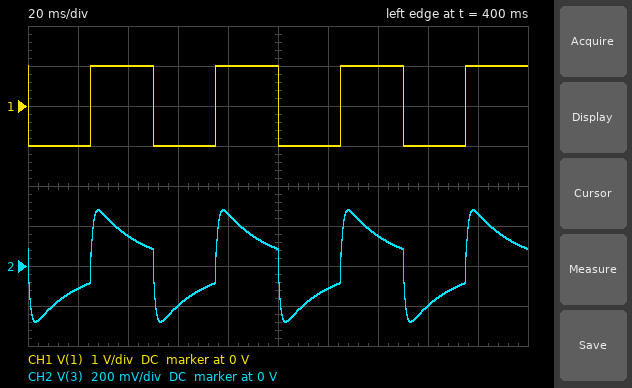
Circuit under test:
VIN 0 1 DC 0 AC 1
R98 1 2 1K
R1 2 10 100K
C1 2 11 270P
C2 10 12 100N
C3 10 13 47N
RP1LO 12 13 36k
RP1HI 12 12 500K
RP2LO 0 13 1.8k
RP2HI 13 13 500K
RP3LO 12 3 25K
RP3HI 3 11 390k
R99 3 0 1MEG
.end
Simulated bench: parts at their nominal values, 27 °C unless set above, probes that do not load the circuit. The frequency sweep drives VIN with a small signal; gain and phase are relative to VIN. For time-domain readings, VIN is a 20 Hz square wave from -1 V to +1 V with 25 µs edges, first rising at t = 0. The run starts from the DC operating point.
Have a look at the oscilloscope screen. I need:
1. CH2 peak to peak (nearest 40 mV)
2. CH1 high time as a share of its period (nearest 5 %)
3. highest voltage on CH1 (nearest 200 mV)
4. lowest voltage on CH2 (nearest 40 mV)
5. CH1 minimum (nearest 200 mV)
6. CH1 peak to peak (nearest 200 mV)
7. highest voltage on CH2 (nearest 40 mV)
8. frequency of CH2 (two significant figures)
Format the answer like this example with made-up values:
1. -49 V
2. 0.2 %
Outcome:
1. 560 mV
2. 50 %
3. 1.0 V
4. -280 mV
5. -1.0 V
6. 2.0 V
7. 280 mV
8. 20 Hz
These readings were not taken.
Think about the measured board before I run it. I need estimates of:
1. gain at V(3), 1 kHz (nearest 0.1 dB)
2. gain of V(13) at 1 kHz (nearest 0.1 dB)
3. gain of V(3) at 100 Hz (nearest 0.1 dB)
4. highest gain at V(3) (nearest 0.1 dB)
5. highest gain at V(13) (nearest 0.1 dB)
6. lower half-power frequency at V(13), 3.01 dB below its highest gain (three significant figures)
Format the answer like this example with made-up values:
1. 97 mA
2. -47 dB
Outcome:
1. -26.5 dB
2. -34.5 dB
3. -15.1 dB
4. -14.1 dB
5. -33.4 dB
6. 83.0 Hz
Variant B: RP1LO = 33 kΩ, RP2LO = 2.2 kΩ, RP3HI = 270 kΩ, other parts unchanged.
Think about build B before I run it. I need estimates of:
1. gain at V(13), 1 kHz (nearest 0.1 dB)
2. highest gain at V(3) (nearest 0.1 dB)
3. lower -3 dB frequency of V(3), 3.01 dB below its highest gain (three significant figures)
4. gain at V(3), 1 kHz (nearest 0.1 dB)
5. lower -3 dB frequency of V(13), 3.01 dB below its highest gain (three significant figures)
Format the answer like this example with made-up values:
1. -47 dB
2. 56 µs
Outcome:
1. -32.9 dB
2. -14.6 dB
3. 8.29 Hz
4. -26.2 dB
5. 189 Hz
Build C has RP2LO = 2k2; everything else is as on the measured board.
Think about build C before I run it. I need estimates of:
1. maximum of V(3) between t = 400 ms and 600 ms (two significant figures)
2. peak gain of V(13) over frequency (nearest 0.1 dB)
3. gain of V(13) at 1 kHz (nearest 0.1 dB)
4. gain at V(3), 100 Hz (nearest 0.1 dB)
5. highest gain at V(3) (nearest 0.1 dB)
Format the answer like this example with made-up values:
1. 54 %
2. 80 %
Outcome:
1. 280 mV
2. -31.7 dB
3. -32.8 dB
4. -15.0 dB
5. -14.0 dB
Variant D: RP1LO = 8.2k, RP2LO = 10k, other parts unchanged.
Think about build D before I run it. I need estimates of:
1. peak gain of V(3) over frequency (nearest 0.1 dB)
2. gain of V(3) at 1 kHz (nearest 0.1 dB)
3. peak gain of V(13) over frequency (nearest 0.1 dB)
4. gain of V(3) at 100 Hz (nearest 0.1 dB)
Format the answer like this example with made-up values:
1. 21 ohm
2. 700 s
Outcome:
1. -16.1 dB
2. -17.9 dB
3. -19.3 dB
4. -17.7 dB
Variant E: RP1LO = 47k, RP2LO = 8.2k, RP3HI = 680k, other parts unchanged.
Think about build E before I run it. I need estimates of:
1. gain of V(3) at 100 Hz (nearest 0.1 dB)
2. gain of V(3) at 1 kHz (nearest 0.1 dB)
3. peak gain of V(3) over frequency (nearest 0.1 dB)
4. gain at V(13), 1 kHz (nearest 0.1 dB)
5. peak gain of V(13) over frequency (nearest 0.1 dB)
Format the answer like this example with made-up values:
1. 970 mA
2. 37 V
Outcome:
1. -12.8 dB
2. -19.7 dB
3. -11.4 dB
4. -22.0 dB
5. -21.5 dB
